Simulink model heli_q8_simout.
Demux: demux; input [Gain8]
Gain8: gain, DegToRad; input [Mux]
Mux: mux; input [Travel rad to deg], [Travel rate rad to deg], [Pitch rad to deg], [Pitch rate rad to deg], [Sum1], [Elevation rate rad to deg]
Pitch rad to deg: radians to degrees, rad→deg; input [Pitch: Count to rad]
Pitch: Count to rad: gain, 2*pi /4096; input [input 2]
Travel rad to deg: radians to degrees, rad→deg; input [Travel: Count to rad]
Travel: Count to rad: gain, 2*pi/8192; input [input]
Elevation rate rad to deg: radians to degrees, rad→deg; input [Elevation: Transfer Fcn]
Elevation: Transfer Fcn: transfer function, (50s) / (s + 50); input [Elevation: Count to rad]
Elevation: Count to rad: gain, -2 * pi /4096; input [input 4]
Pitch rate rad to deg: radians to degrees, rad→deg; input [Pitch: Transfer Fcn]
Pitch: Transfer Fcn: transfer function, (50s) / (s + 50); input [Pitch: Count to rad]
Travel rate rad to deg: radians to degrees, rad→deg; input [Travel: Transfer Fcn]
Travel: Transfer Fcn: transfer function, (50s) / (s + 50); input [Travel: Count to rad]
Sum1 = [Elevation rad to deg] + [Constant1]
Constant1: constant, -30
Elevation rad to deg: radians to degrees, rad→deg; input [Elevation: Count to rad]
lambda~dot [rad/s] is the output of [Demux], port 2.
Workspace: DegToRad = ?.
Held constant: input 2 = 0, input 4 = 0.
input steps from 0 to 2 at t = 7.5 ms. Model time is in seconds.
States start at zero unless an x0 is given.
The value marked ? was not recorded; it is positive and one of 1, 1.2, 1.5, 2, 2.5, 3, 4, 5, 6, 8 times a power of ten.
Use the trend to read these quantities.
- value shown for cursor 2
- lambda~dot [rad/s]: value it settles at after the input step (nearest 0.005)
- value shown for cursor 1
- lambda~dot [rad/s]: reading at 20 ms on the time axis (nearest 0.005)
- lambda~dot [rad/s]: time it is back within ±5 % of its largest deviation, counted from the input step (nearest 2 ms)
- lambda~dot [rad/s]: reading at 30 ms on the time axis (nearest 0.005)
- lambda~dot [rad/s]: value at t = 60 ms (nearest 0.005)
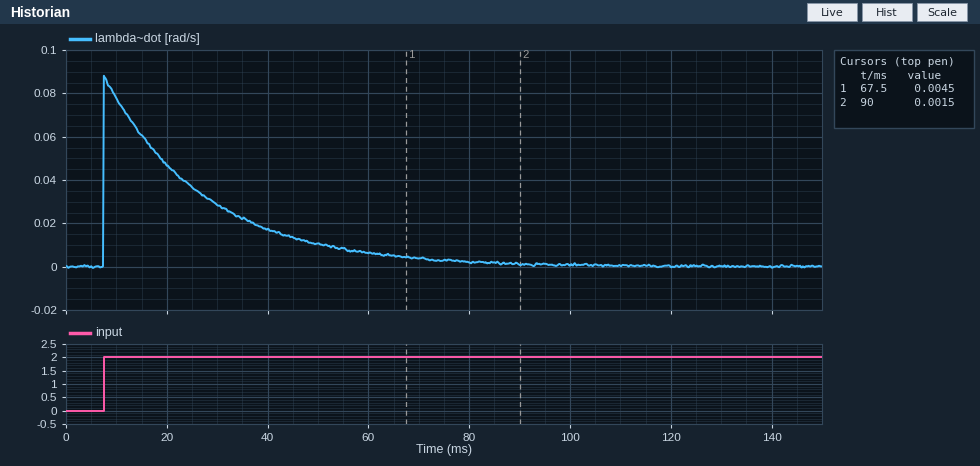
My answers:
0.0015
0.000
0.0045
0.045
60 ms
0.030
0.005
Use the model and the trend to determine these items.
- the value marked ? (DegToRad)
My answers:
0.02
